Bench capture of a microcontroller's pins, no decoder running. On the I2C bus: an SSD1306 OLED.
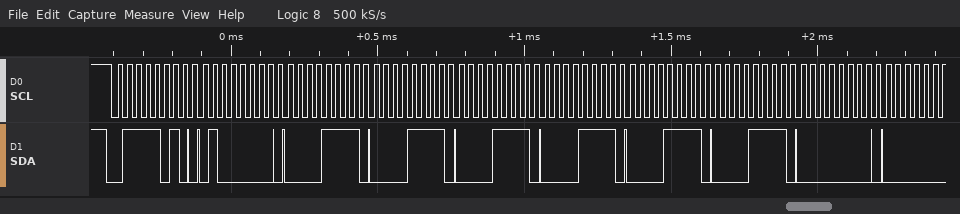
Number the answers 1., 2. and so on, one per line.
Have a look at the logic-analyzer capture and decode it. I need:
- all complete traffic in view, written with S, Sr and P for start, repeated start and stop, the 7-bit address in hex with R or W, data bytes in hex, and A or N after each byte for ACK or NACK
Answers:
1. S 3DW A 40 A 0F A 0F A 0F A 0F A 0F A 0F A 00 A
